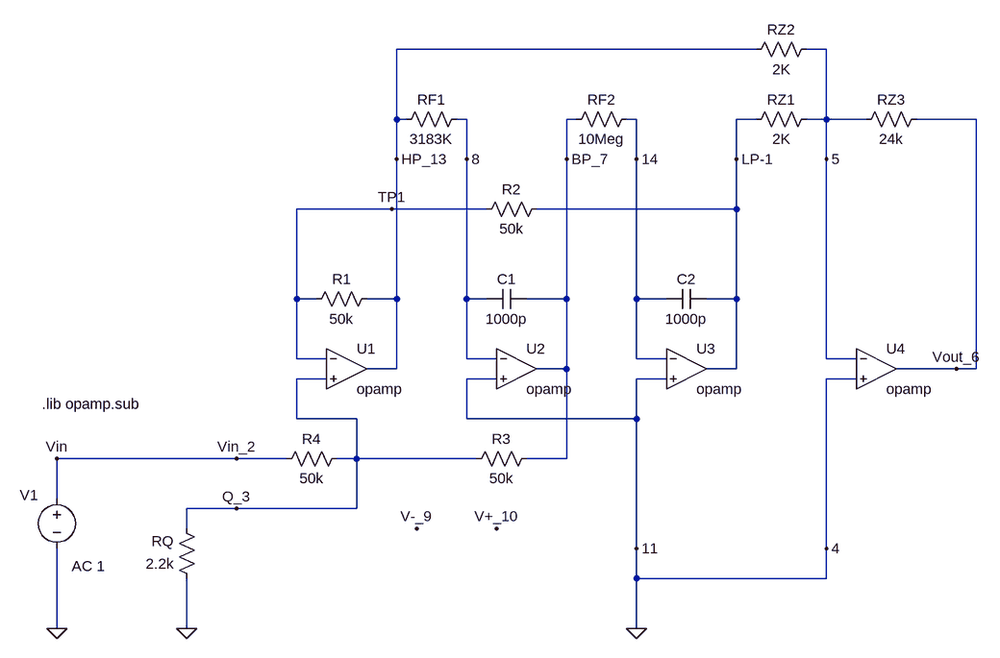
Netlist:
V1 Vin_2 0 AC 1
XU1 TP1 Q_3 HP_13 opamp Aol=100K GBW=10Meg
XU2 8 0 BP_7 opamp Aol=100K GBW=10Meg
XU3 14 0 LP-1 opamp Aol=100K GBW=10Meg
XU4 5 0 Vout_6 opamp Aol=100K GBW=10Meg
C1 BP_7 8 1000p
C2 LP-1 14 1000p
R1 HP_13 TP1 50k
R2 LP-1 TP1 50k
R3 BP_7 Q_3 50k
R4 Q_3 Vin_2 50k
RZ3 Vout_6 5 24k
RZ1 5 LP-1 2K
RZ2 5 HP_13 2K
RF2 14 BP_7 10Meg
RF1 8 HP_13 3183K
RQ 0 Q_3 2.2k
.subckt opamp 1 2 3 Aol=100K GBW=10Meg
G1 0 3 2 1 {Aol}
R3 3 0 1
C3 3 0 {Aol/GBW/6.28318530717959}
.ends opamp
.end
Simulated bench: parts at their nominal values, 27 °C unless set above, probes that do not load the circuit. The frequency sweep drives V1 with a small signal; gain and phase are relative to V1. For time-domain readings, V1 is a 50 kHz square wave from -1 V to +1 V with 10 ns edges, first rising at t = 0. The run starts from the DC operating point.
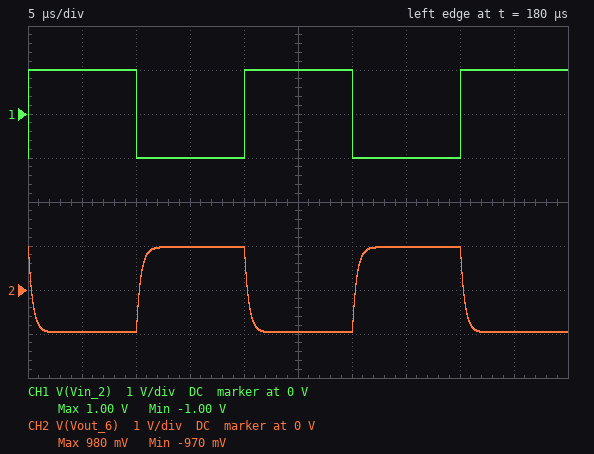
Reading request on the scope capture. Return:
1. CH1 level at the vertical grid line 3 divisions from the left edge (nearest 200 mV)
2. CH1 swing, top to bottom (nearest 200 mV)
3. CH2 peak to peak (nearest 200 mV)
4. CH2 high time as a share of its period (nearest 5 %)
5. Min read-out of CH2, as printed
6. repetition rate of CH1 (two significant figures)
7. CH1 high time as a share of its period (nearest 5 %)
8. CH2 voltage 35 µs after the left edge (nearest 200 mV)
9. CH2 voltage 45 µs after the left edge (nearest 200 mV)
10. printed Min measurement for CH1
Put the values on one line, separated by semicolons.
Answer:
-1.0 V; 2.0 V; 2.0 V; 50 %; -970 mV; 50 kHz; 50 %; 1.0 V; -1.0 V; -1.00 V
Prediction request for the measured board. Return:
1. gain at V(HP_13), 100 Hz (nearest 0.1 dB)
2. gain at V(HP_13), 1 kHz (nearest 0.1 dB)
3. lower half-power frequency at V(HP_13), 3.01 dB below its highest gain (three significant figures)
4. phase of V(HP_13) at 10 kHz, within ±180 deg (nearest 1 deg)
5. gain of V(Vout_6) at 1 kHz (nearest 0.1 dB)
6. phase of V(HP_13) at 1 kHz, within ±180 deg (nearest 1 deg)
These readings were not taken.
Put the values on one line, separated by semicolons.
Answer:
-21.1 dB; -21.8 dB; 26.5 Hz; 0 deg; -0.3 dB; 0 deg
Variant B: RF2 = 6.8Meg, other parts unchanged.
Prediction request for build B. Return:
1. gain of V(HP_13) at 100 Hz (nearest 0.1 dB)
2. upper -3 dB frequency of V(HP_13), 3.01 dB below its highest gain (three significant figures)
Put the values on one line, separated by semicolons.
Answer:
-20.8 dB; 36.6 Hz
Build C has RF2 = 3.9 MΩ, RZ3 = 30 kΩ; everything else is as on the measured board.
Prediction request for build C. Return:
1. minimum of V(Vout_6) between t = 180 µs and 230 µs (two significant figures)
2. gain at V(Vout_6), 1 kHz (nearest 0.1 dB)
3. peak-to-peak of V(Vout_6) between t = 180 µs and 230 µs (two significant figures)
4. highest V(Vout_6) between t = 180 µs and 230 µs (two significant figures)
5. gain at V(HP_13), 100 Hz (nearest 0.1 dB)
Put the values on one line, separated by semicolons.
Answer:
-1.2 V; 1.7 dB; 2.4 V; 1.2 V; -19.9 dB
